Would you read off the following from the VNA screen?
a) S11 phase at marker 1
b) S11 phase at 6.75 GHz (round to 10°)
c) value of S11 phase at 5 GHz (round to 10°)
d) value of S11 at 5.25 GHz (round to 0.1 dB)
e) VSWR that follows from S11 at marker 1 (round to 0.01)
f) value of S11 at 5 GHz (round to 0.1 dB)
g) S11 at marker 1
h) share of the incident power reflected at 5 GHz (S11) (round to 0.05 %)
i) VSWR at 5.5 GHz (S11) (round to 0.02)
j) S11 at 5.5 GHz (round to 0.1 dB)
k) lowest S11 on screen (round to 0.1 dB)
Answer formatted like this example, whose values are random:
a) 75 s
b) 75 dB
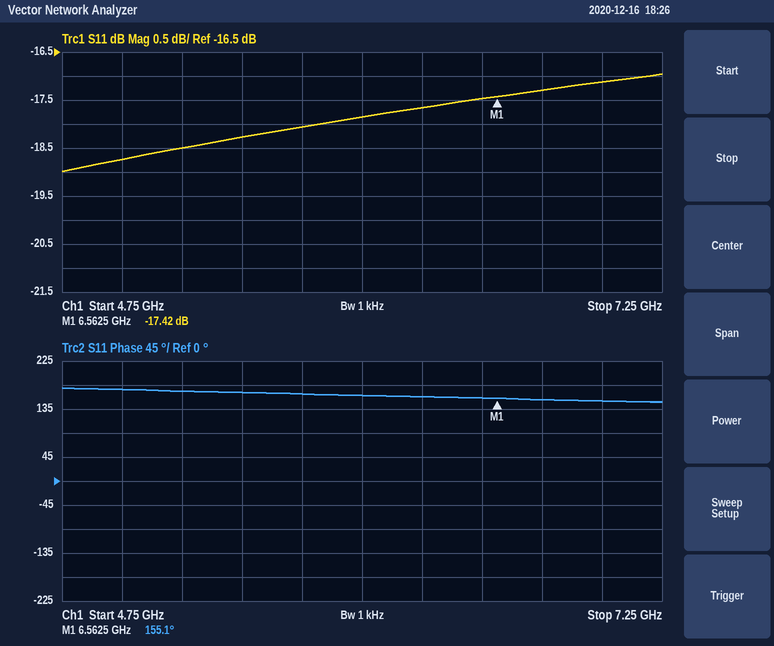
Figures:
a) 155.1°
b) 150°
c) 170°
d) -18.5 dB
e) 1.31
f) -18.7 dB
g) -17.42 dB
h) 1.35 %
i) 1.28
j) -18.3 dB
k) -19.0 dB
